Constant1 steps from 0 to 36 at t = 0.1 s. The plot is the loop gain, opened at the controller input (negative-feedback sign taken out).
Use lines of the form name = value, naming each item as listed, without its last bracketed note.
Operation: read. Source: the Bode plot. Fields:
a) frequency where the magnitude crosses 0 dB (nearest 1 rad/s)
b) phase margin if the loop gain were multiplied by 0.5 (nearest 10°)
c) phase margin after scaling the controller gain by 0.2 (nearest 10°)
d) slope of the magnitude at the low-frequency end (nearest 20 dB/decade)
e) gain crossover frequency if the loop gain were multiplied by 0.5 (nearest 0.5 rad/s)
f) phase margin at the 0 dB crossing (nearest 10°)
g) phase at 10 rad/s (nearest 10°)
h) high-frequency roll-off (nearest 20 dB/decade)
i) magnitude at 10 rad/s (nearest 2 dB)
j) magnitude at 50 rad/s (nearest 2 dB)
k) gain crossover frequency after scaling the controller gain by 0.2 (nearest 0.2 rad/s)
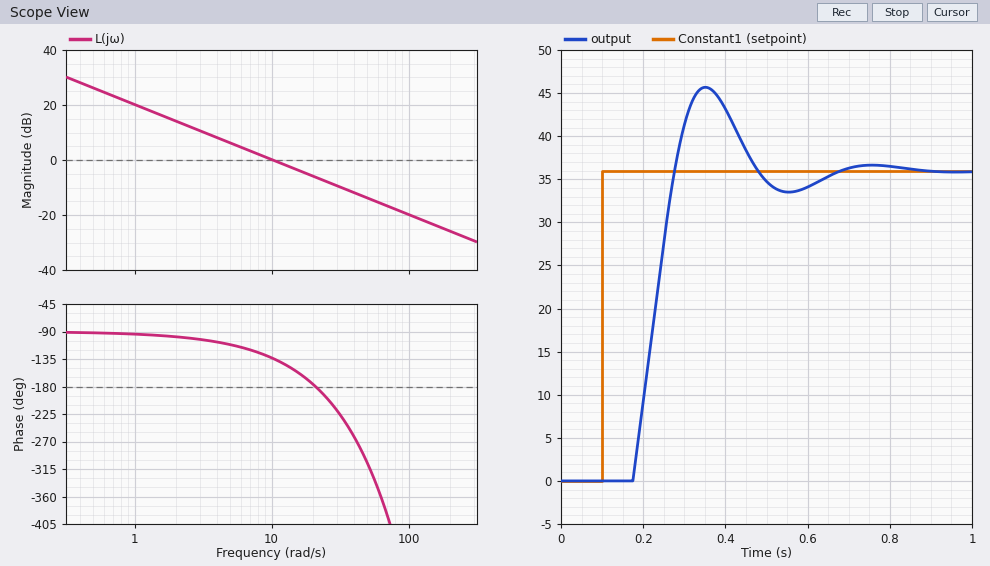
frequency where the magnitude crosses 0 dB = 10 rad/s
phase margin if the loop gain were multiplied by 0.5 = 70°
phase margin after scaling the controller gain by 0.2 = 80°
slope of the magnitude at the low-frequency end = -20 dB/decade
gain crossover frequency if the loop gain were multiplied by 0.5 = 5.0 rad/s
phase margin at the 0 dB crossing = 50°
phase at 10 rad/s = -130°
high-frequency roll-off = -20 dB/decade
magnitude at 10 rad/s = 0 dB
magnitude at 50 rad/s = -14 dB
gain crossover frequency after scaling the controller gain by 0.2 = 2.0 rad/s
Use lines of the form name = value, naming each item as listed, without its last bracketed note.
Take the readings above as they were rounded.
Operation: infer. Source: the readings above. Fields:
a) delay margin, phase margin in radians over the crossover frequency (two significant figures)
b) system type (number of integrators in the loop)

delay margin, phase margin in radians over the crossover frequency = 0.087 s
system type = 1
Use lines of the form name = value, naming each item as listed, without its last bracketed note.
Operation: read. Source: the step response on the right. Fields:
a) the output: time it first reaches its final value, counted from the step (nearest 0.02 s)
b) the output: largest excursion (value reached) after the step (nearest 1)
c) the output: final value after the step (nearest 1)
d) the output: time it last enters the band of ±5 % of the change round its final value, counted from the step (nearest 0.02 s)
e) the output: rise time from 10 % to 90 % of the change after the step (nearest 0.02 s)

the output: time it first reaches its final value, counted from the step = 0.18 s
the output: largest excursion (value reached) after the step = 46
the output: final value after the step = 36
the output: time it last enters the band of ±5 % of the change round its final value, counted from the step = 0.50 s
the output: rise time from 10 % to 90 % of the change after the step = 0.08 s
